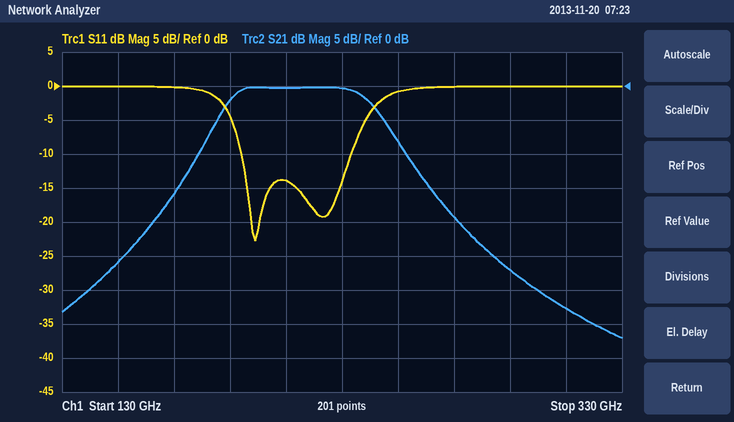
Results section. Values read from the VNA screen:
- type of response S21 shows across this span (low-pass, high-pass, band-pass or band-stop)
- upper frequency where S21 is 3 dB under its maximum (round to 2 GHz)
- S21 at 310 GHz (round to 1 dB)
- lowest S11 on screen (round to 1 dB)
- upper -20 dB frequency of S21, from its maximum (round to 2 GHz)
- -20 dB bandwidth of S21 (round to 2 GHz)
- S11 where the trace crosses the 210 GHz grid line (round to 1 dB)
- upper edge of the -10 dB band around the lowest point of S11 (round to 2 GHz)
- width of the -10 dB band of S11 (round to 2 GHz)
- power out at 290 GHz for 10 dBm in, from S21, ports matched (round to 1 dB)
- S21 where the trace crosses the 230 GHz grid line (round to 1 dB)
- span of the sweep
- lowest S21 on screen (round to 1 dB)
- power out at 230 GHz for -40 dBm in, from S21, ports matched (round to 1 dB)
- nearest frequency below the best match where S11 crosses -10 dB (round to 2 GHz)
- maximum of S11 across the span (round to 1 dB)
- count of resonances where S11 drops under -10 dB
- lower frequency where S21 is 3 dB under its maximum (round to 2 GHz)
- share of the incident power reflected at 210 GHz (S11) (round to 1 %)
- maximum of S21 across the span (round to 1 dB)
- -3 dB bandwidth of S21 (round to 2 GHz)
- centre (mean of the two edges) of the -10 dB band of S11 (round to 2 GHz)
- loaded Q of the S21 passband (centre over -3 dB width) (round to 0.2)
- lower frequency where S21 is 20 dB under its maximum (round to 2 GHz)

band-pass
242 GHz
-33 dB
-23 dB
272 GHz
110 GHz
-14 dB
234 GHz
40 GHz
-17 dBm
0 dB
200 GHz
-37 dB
-40 dBm
194 GHz
0 dB
2
188 GHz
4 %
0 dB
54 GHz
214 GHz
4.0
162 GHz
